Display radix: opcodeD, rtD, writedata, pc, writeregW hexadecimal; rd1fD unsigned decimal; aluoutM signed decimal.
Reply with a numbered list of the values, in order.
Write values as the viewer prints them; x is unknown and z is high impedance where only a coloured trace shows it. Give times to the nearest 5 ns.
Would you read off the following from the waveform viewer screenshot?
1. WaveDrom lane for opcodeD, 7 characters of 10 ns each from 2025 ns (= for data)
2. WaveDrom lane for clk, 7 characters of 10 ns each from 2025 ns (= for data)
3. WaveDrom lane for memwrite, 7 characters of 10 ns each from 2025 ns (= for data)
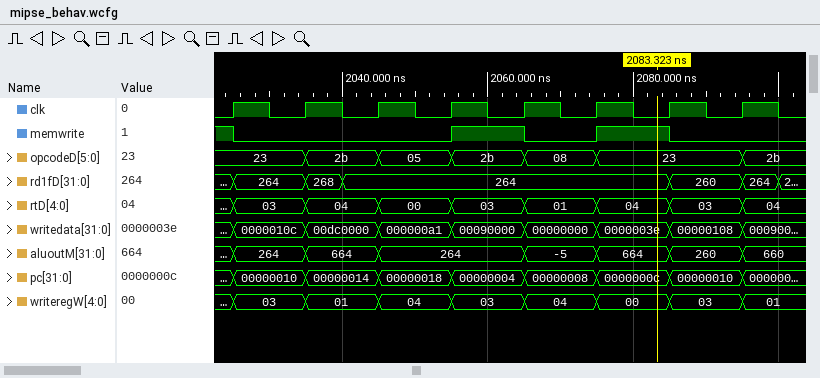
1. {name: 'opcodeD', wave: '======.', data: '23 2b 05 2b 08 23'}
2. {name: 'clk', wave: 'p......'}
3. {name: 'memwrite', wave: '0..1010'}
